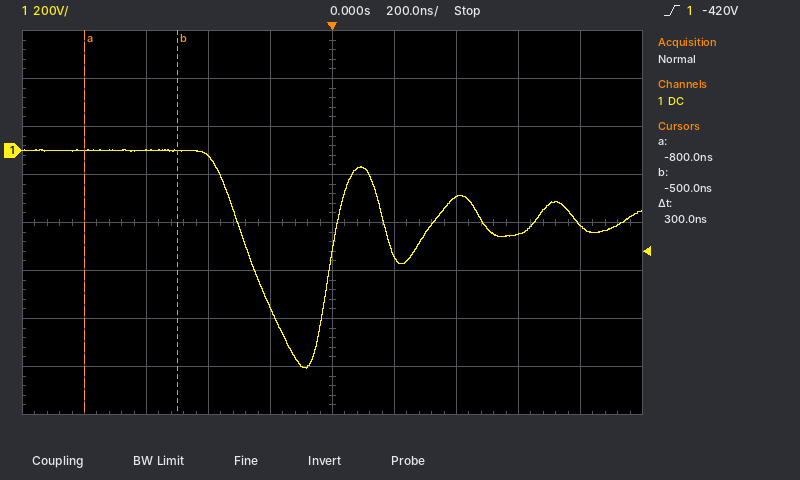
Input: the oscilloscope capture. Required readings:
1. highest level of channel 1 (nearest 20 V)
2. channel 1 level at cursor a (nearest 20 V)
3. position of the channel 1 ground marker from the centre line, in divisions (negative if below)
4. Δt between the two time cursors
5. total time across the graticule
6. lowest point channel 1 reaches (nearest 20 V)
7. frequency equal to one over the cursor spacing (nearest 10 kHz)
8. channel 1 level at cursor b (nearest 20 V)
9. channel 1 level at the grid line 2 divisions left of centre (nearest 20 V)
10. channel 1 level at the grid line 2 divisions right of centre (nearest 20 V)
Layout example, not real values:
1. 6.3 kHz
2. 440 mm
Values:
1. 0 V
2. 0 V
3. +1.5 div
4. 300 ns
5. 2 µs
6. -900 V
7. 3.33 MHz
8. 0 V
9. -20 V
10. -200 V
